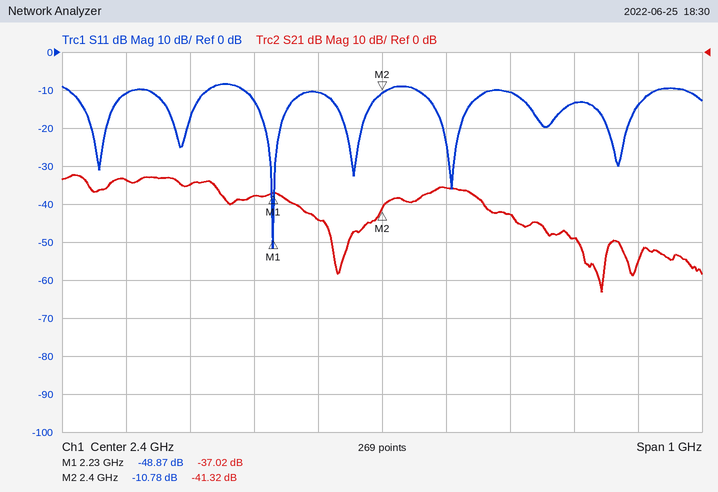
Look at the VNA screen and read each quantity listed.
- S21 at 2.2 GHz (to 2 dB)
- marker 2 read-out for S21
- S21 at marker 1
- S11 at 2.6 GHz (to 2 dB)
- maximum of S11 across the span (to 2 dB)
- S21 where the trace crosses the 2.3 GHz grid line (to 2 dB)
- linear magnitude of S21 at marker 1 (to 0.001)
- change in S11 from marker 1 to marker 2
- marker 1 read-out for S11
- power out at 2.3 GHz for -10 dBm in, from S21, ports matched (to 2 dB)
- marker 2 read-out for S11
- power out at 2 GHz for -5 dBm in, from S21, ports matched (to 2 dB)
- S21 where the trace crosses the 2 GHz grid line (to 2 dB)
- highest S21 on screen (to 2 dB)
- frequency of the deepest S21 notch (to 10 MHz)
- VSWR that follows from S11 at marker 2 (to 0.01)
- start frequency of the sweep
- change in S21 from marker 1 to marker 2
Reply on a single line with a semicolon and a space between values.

-38 dB; -41.32 dB; -37.02 dB; -10 dB; -8 dB; -44 dB; 0.014; 38.09 dB; -48.87 dB; -54 dBm; -10.78 dB; -38 dBm; -34 dB; -32 dB; 2.74 GHz; 1.81; 1.9 GHz; -4.30 dB
